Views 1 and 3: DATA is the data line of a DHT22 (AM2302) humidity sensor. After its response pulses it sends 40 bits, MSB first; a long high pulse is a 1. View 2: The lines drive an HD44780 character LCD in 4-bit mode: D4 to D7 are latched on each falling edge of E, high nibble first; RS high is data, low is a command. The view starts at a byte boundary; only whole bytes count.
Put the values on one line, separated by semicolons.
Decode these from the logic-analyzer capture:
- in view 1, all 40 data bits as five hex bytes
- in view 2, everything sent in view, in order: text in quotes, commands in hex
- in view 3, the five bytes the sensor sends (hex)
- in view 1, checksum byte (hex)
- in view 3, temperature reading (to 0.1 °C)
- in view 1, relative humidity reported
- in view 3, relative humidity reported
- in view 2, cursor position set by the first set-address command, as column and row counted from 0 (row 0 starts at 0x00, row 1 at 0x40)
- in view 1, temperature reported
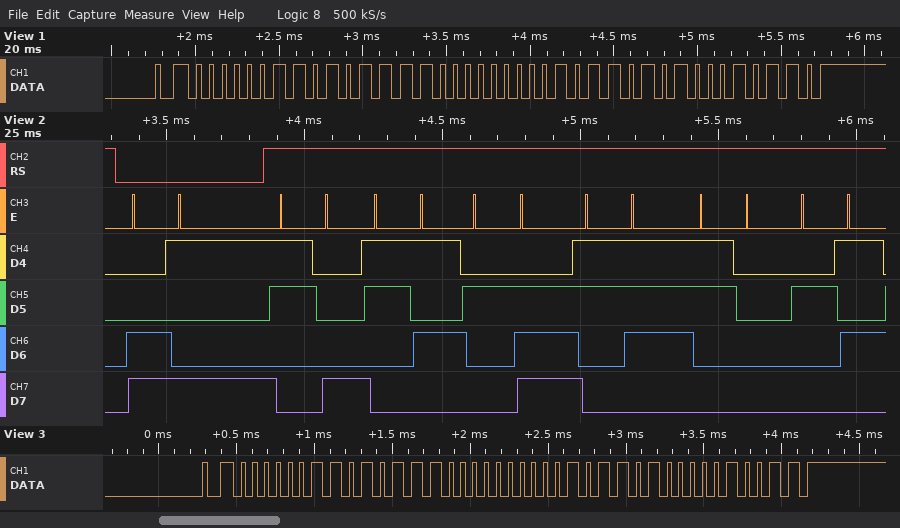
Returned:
03 5E 00 B5 16; 0xC9 "85.70%"; 03 5C 00 B4 13; 0x16; 18.0 °C; 86.2 %; 86.0 %; column 9, row 1; 18.1 °C
